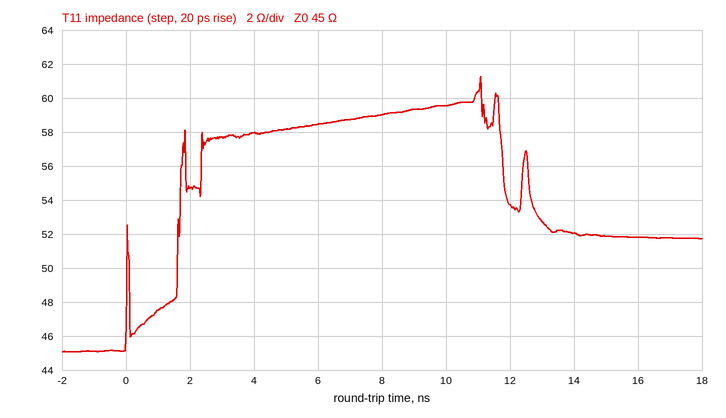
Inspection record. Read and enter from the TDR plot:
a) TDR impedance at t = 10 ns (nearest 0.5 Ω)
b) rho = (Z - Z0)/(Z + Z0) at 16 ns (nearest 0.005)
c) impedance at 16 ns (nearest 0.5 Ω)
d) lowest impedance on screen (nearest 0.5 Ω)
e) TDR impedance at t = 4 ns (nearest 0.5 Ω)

59.5 Ω
+0.070
52.0 Ω
45.0 Ω
58.0 Ω
